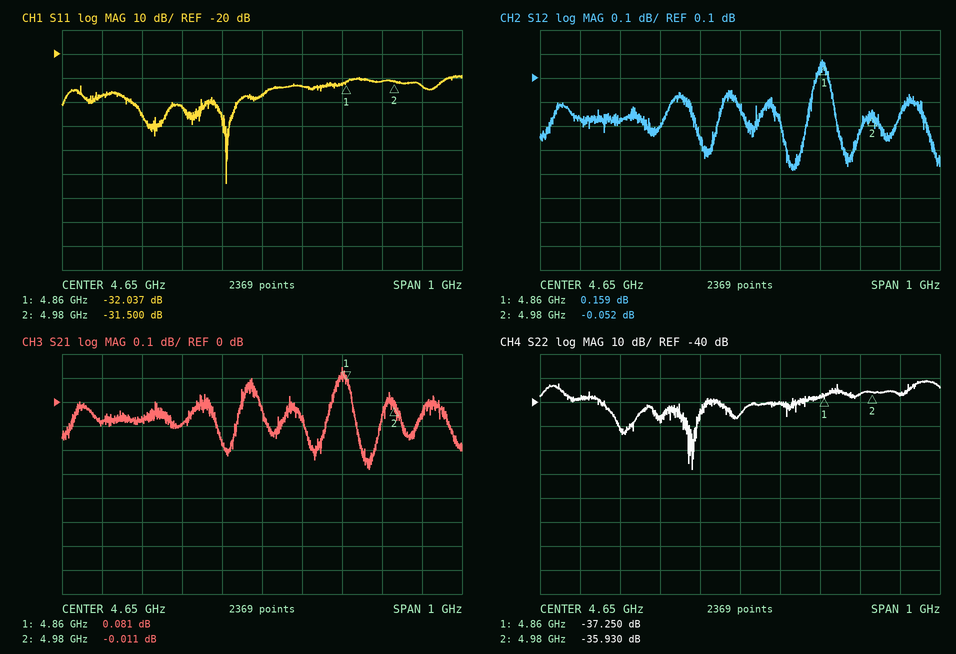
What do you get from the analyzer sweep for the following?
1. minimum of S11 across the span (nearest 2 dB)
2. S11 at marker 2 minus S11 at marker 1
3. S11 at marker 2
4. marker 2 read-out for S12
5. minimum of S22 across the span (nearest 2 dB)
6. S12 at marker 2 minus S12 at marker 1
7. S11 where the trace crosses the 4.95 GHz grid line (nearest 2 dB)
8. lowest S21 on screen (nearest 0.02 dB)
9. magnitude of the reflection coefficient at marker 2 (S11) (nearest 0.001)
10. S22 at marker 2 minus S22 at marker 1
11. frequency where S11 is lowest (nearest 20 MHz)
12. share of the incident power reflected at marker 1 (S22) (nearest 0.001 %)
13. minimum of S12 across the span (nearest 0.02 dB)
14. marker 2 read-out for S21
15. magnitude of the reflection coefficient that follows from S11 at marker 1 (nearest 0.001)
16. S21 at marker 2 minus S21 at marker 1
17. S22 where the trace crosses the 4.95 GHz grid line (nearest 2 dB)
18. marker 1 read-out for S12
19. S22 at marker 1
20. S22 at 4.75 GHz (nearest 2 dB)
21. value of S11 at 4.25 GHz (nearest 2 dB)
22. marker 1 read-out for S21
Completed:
-74 dB
0.537 dB
-31.500 dB
-0.052 dB
-68 dB
-0.211 dB
-32 dB
-0.28 dB
0.027
1.320 dB
4.56 GHz
0.019 %
-0.28 dB
-0.011 dB
0.025
-0.092 dB
-36 dB
0.159 dB
-37.250 dB
-40 dB
-38 dB
0.081 dB
